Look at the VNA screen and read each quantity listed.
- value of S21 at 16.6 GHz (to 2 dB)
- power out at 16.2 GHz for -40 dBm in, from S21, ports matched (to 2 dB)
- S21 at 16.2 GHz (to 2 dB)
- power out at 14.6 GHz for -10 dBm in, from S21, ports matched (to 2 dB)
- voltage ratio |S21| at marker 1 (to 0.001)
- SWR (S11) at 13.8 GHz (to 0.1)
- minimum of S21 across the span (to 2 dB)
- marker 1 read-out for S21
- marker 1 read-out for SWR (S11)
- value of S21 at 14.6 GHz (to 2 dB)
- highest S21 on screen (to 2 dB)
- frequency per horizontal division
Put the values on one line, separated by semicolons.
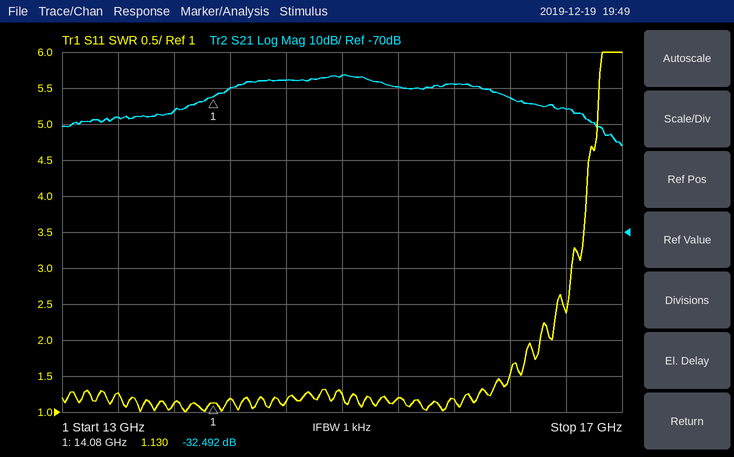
-36 dB; -72 dBm; -32 dB; -38 dBm; 0.024; 1.1; -46 dB; -32.492 dB; 1.130; -28 dB; -26 dB; 400 MHz
